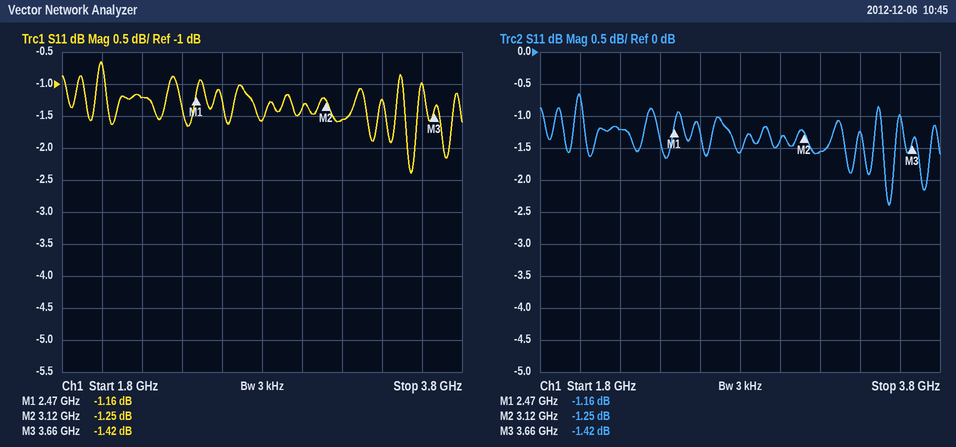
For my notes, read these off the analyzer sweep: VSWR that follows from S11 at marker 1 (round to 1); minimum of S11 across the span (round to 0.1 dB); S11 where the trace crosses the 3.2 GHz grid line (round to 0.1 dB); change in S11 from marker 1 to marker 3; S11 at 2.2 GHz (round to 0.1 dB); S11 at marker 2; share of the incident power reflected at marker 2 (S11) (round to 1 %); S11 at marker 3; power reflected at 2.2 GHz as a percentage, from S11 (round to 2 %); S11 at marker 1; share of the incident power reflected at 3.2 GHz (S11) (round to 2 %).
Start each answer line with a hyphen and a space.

- 15
- -2.4 dB
- -1.6 dB
- -0.26 dB
- -1.2 dB
- -1.25 dB
- 75 %
- -1.42 dB
- 76 %
- -1.16 dB
- 70 %
